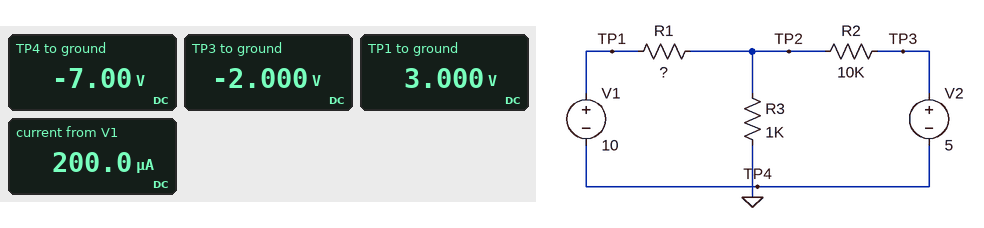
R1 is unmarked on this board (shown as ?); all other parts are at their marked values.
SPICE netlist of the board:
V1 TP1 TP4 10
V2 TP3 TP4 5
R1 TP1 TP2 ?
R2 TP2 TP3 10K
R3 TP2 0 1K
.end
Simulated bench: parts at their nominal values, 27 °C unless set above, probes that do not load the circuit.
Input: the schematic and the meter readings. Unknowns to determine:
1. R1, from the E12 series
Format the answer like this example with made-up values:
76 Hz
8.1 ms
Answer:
15 kΩ
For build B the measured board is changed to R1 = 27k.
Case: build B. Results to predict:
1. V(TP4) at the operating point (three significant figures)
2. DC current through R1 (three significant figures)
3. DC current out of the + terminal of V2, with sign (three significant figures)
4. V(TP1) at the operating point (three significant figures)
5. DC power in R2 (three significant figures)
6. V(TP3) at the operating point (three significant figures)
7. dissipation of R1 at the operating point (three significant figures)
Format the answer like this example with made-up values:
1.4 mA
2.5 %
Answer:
-6.35 V
135 µA
-135 µA
3.65 V
183 µW
-1.35 V
493 µW
